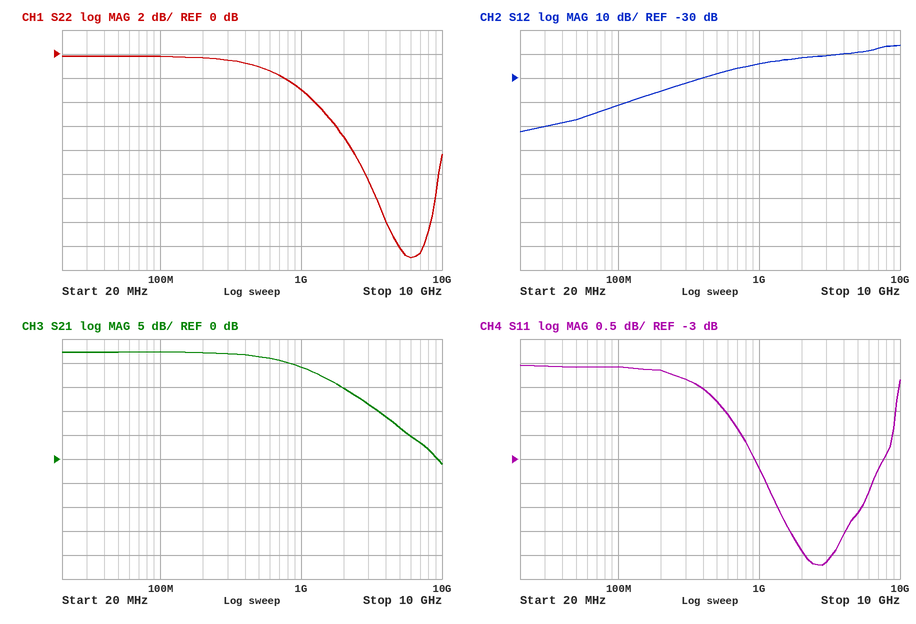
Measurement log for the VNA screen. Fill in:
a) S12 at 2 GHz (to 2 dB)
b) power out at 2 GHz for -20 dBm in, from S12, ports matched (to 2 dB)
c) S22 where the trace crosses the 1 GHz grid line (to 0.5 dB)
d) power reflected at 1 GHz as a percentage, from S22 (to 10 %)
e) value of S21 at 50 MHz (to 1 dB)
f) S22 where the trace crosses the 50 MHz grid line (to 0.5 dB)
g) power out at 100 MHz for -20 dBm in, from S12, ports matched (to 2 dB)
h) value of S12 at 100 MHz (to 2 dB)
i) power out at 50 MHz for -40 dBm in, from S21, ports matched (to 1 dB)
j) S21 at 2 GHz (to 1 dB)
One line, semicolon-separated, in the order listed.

-22 dB; -42 dBm; -3.0 dB; 50 %; 22 dB; 0.0 dB; -62 dBm; -42 dB; -18 dBm; 15 dB
